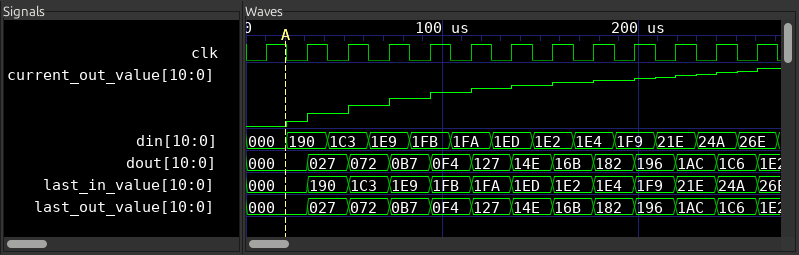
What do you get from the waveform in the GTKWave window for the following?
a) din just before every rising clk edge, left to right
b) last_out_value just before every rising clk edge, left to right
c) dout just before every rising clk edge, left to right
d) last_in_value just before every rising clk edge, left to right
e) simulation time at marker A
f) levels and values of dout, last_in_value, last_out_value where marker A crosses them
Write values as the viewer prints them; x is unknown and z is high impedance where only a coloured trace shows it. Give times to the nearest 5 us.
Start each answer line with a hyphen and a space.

- 000, 190, 1C3, 1E9, 1FB, 1FA, 1ED, 1E2, 1E4, 1F9, 21E, 24A, 26E
- 000, 000, 027, 072, 0B7, 0F4, 127, 14E, 16B, 182, 196, 1AC, 1C6
- 000, 000, 027, 072, 0B7, 0F4, 127, 14E, 16B, 182, 196, 1AC, 1C6
- 000, 000, 190, 1C3, 1E9, 1FB, 1FA, 1ED, 1E2, 1E4, 1F9, 21E, 24A
- 20 us
- dout=000, last_in_value=000, last_out_value=000
